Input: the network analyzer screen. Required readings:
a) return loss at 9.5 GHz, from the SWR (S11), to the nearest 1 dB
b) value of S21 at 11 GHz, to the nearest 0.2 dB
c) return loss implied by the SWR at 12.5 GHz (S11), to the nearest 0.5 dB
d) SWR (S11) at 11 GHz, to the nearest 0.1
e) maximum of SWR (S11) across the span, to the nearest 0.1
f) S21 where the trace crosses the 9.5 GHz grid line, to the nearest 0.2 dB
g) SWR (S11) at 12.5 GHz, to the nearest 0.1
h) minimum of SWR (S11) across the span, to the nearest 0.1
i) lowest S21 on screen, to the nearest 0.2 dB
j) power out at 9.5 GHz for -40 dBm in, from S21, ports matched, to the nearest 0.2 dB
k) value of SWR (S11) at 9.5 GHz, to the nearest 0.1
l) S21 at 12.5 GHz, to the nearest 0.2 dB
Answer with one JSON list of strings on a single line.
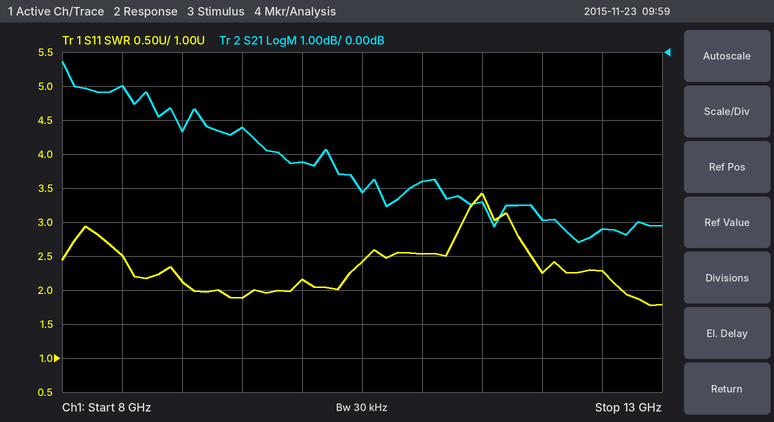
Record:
["10 dB", "-3.8 dB", "8.0 dB", "2.5", "3.4", "-2.2 dB", "2.3", "1.8", "-5.6 dB", "-42.2 dBm", "1.9", "-5.2 dB"]
